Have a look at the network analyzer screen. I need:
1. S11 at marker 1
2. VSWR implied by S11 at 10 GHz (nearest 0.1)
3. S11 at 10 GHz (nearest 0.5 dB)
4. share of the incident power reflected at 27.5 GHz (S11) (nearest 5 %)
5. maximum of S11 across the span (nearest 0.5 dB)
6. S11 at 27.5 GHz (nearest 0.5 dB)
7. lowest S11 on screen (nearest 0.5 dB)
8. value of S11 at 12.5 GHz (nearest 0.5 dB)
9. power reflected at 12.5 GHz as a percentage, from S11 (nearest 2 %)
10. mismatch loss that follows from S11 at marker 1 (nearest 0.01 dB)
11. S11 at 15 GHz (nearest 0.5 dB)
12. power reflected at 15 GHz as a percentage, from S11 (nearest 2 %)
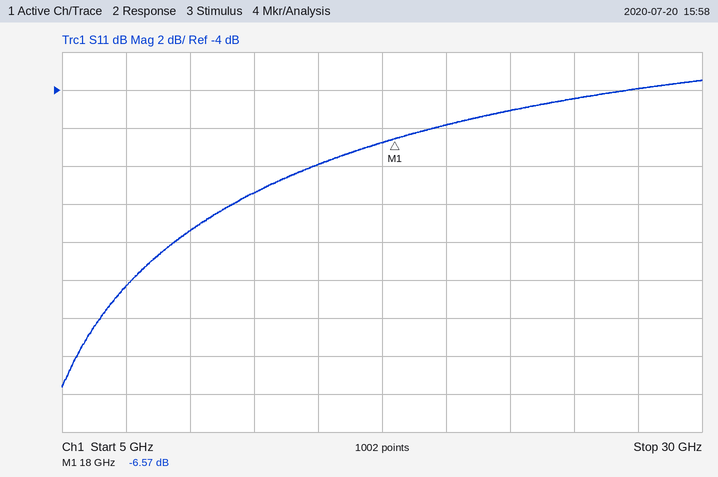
-6.57 dB
1.7
-11.5 dB
40 %
-3.5 dB
-4.0 dB
-19.5 dB
-9.5 dB
12 %
1.08 dB
-8.0 dB
16 %
